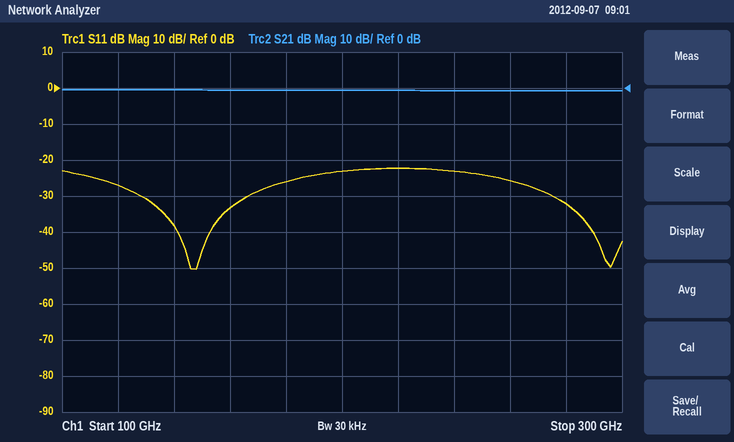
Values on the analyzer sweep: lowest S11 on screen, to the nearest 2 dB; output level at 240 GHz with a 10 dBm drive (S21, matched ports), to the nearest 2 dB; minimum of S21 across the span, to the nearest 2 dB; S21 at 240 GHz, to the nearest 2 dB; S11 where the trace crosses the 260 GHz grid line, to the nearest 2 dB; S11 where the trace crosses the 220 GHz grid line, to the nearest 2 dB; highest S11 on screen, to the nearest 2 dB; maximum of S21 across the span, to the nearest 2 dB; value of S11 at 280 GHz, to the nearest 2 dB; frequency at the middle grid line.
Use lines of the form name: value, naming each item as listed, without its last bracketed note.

lowest S11 on screen, to the nearest 2 dB: -50 dB
output level at 240 GHz with a 10 dBm drive (S21, matched ports), to the nearest 2 dB: 10 dBm
minimum of S21 across the span, to the nearest 2 dB: 0 dB
S21 at 240 GHz, to the nearest 2 dB: 0 dB
S11 where the trace crosses the 260 GHz grid line, to the nearest 2 dB: -26 dB
S11 where the trace crosses the 220 GHz grid line, to the nearest 2 dB: -22 dB
highest S11 on screen, to the nearest 2 dB: -22 dB
maximum of S21 across the span, to the nearest 2 dB: 0 dB
value of S11 at 280 GHz, to the nearest 2 dB: -32 dB
frequency at the middle grid line: 200 GHz
